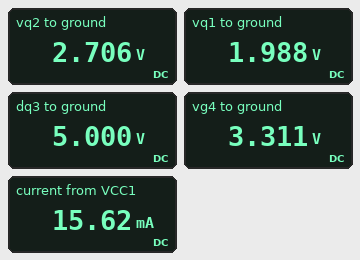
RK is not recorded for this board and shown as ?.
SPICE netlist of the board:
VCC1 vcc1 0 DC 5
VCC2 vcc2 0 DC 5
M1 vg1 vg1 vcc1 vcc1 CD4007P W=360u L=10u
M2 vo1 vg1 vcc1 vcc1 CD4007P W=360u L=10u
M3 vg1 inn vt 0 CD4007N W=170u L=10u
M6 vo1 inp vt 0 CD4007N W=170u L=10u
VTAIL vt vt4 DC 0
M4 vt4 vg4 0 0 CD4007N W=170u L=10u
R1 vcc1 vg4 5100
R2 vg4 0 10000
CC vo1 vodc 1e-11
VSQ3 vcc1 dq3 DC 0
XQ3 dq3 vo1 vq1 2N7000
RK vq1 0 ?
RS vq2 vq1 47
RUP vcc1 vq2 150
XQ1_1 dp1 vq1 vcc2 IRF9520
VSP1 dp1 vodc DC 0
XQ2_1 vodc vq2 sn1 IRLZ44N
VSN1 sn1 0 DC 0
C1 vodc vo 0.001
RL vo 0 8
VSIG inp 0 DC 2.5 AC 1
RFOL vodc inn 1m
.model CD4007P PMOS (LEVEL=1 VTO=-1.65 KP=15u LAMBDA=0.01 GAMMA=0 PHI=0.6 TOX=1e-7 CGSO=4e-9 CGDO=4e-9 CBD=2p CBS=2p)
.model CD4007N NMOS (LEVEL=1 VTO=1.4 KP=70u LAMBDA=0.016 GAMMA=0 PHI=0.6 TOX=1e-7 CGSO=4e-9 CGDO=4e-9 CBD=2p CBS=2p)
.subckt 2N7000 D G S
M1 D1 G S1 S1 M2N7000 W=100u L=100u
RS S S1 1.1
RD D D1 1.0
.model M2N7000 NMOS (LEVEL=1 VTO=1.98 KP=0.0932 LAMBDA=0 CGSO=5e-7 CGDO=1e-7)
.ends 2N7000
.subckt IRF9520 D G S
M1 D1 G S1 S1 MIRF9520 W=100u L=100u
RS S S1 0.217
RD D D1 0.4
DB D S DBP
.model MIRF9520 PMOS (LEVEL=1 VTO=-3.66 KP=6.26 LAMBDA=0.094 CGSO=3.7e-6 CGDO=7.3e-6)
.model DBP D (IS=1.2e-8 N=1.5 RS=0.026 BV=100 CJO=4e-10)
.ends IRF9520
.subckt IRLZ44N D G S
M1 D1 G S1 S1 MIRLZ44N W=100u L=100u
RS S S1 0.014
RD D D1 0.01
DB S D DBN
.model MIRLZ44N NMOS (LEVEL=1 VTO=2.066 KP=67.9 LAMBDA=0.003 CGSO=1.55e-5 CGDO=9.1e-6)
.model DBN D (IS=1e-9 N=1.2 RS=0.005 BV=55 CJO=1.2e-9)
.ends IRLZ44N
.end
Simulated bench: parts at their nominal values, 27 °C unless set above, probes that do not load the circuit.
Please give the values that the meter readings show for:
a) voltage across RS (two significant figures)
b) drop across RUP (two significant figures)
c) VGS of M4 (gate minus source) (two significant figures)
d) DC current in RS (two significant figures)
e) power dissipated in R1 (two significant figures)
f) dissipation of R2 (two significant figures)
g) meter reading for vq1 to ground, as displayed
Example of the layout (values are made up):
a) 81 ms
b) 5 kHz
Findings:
a) 720 mV
b) 2.3 V
c) 3.3 V
d) 15 mA
e) 560 µW
f) 1.1 mW
g) 1.988 V
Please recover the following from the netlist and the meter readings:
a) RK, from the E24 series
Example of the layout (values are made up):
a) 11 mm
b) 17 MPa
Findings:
a) 130 Ω
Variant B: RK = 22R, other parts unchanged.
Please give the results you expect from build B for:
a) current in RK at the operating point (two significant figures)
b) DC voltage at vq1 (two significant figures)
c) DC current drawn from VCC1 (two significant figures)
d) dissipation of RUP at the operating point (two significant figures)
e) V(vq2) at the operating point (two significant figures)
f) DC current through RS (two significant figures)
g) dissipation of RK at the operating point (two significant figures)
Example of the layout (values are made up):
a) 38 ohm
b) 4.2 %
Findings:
a) 55 mA
b) 1.2 V
c) 56 mA
d) 56 mW
e) 2.1 V
f) 19 mA
g) 66 mW
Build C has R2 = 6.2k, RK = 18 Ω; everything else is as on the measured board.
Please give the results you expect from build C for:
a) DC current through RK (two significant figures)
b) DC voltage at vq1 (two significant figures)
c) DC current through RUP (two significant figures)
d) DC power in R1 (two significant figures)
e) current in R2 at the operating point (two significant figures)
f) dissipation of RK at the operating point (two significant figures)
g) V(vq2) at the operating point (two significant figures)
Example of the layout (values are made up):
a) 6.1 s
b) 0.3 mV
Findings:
a) 67 mA
b) 1.2 V
c) 19 mA
d) 1.0 mW
e) 440 µA
f) 80 mW
g) 2.1 V
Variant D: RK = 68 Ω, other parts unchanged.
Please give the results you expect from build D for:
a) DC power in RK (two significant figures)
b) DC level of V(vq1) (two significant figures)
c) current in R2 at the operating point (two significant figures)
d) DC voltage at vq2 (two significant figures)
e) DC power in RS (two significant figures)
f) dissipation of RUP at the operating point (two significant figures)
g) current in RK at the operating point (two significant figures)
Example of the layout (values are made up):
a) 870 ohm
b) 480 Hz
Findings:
a) 24 mW
b) 1.3 V
c) 330 µA
d) 2.2 V
e) 17 mW
f) 53 mW
g) 19 mA
